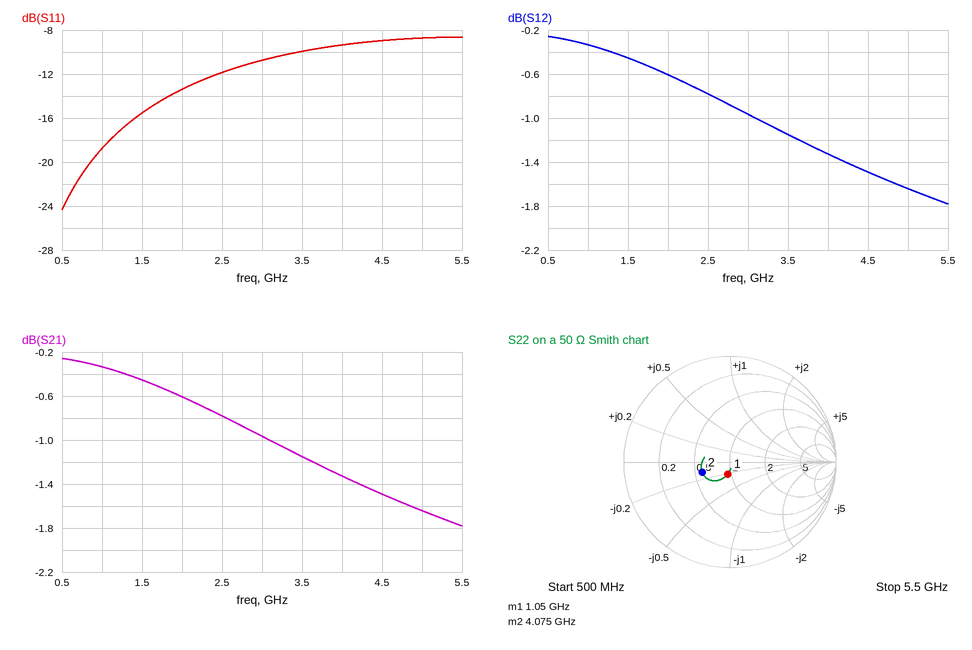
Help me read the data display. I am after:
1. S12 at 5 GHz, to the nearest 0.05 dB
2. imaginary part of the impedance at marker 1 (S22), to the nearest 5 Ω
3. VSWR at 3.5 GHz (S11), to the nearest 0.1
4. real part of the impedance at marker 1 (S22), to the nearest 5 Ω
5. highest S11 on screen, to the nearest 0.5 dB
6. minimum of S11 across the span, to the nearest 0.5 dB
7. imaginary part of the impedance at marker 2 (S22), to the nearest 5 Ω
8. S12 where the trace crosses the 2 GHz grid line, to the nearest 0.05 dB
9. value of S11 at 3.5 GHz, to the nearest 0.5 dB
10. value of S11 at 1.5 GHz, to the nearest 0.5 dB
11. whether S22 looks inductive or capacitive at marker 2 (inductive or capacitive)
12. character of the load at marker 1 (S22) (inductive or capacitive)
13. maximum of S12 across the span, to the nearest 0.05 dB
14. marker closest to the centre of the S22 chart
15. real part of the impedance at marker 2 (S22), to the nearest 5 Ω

-1.65 dB
-10 Ω
1.9
45 Ω
-8.5 dB
-24.5 dB
-5 Ω
-0.60 dB
-10.0 dB
-15.5 dB
capacitive
capacitive
-0.25 dB
marker 1
30 Ω
